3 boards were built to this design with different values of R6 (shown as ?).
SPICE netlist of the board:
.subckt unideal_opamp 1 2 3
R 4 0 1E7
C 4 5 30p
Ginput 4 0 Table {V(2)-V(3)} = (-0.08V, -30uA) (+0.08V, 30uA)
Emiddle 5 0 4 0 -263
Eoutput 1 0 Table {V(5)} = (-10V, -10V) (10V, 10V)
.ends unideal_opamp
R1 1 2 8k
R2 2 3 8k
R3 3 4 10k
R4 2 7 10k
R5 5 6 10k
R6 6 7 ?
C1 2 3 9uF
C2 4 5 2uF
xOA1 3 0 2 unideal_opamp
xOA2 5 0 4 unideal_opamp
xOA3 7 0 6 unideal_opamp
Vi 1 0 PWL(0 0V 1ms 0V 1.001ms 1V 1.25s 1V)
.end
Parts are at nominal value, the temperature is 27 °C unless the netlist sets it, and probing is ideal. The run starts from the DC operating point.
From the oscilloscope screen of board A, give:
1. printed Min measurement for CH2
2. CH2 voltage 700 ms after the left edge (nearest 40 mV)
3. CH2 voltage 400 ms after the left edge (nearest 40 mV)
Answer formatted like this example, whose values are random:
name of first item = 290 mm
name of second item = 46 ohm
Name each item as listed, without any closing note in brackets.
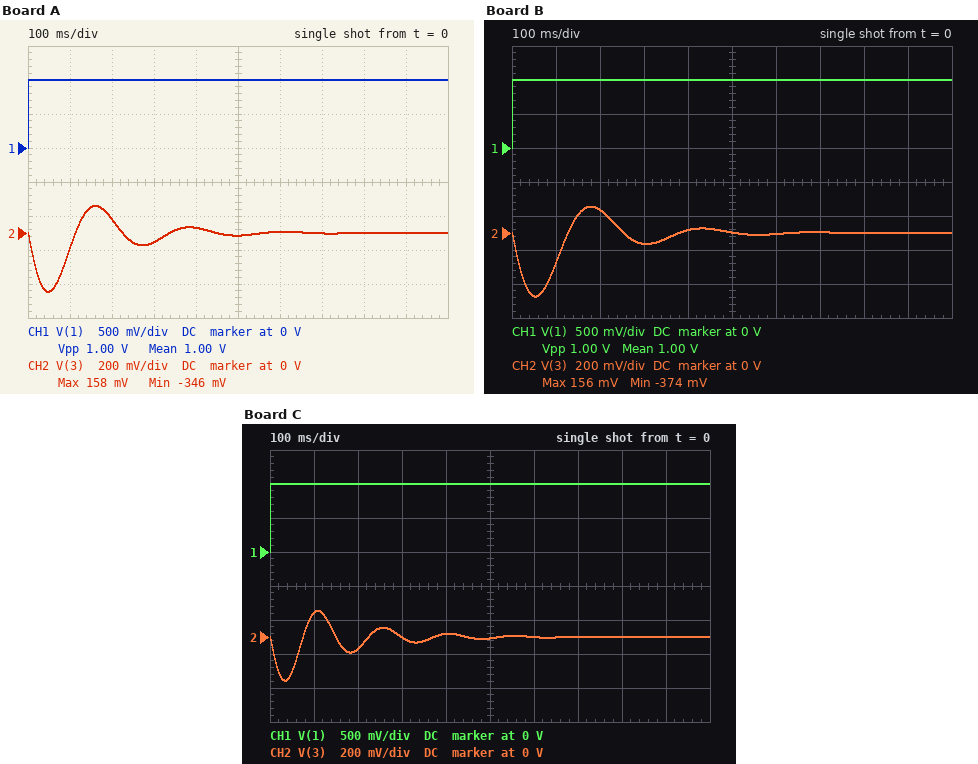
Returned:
printed Min measurement for CH2 = -346 mV
CH2 voltage 700 ms after the left edge = 0 V
CH2 voltage 400 ms after the left edge = 40 mV
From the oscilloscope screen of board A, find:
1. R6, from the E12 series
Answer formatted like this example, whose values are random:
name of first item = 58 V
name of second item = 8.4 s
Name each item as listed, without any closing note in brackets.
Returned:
R6, from the E12 series = 15 kΩ
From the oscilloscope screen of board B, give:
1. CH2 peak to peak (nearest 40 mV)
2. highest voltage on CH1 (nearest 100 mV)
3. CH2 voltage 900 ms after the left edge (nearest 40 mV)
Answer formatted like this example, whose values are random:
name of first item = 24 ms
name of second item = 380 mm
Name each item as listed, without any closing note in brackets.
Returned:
CH2 peak to peak = 520 mV
highest voltage on CH1 = 1.0 V
CH2 voltage 900 ms after the left edge = 0 V
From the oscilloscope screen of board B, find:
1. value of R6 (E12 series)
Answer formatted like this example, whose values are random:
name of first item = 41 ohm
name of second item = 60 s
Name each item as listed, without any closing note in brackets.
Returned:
value of R6 = 12 kΩ
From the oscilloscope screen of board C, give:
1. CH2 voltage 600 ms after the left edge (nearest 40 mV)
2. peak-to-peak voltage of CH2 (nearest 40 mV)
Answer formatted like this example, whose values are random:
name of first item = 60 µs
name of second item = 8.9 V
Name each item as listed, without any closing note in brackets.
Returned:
CH2 voltage 600 ms after the left edge = 0 V
peak-to-peak voltage of CH2 = 400 mV
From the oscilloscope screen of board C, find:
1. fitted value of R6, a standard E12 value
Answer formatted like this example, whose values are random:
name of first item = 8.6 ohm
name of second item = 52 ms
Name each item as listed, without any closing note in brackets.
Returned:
fitted value of R6, a standard E12 value = 33 kΩ
